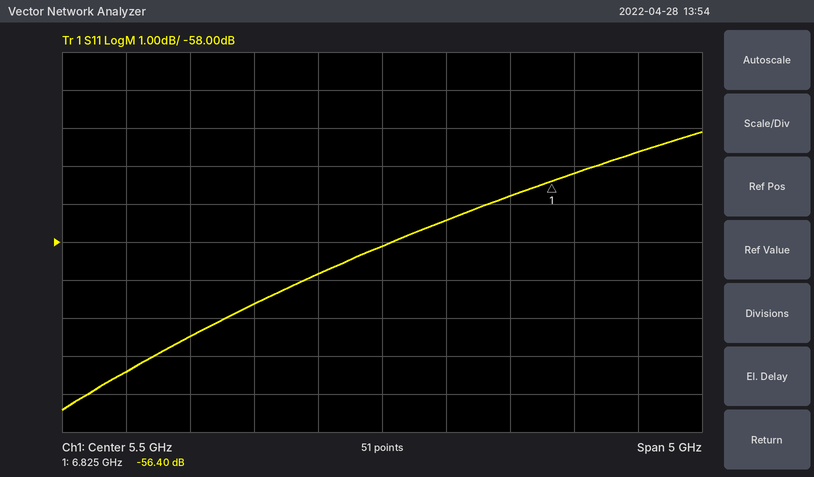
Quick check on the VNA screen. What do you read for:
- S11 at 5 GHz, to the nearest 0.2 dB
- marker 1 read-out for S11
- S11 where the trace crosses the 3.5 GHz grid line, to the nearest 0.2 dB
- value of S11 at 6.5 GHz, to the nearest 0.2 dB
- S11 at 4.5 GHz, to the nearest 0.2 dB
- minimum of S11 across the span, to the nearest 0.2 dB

-58.8 dB
-56.40 dB
-61.4 dB
-56.8 dB
-59.6 dB
-62.4 dB
